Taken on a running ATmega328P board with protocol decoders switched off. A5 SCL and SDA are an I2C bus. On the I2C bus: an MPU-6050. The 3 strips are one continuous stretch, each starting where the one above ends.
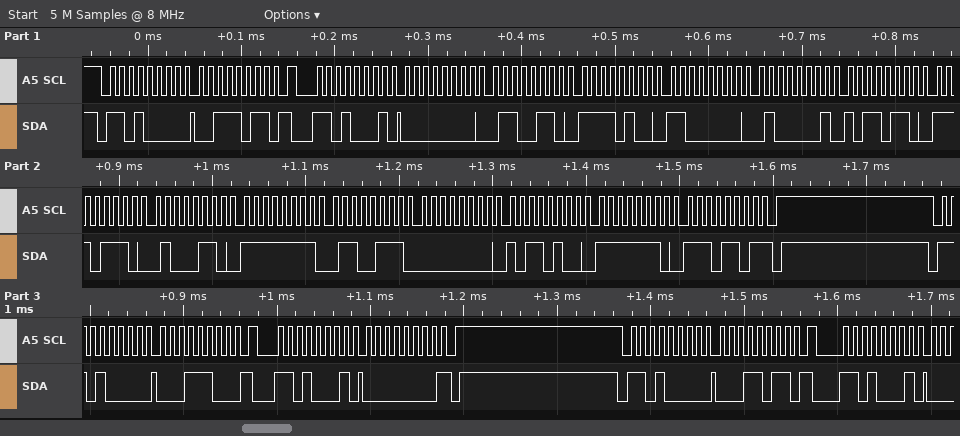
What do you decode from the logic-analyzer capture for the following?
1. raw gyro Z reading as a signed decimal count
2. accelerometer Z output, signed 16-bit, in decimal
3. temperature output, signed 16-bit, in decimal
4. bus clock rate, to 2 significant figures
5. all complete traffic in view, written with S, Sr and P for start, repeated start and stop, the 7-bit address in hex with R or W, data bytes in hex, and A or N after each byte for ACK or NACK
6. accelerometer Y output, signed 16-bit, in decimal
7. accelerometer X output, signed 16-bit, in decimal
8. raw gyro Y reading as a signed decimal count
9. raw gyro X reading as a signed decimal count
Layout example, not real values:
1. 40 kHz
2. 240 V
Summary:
1. -275
2. 16822
3. -4538
4. 100 kHz
5. S 68W A 3B A Sr 68R A 00 A 66 A F4 A C0 A 41 A B6 A EE A 46 A FF A 67 A 00 A B4 A FE A ED N P S 68W A 1C A Sr 68R A 00 N P S 68W A 1B A Sr 68R A
6. -2880
7. 102
8. 180
9. -153
